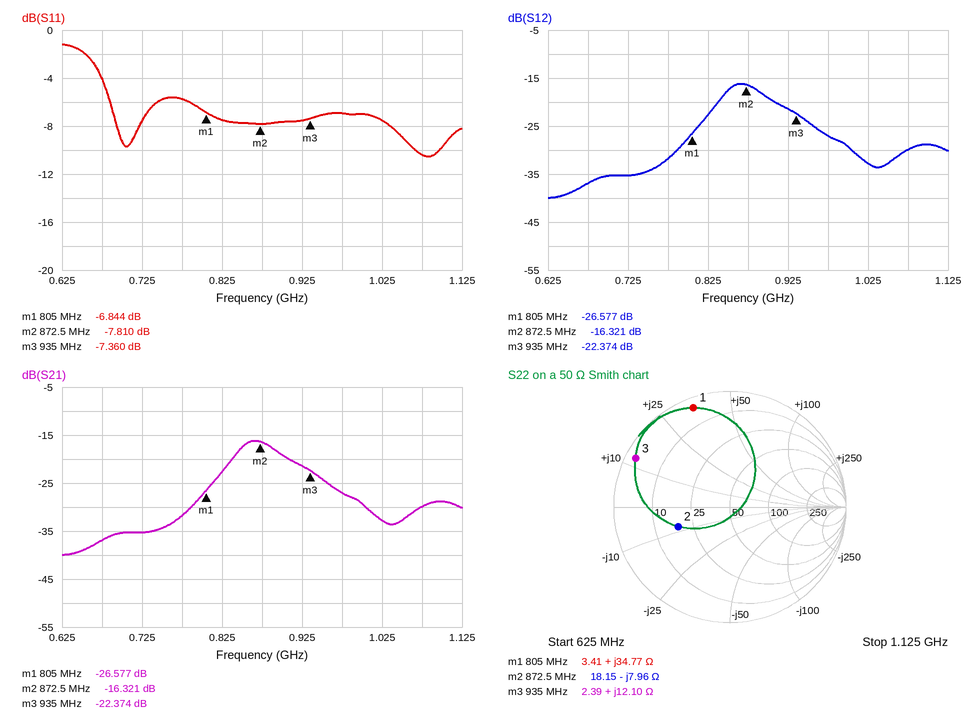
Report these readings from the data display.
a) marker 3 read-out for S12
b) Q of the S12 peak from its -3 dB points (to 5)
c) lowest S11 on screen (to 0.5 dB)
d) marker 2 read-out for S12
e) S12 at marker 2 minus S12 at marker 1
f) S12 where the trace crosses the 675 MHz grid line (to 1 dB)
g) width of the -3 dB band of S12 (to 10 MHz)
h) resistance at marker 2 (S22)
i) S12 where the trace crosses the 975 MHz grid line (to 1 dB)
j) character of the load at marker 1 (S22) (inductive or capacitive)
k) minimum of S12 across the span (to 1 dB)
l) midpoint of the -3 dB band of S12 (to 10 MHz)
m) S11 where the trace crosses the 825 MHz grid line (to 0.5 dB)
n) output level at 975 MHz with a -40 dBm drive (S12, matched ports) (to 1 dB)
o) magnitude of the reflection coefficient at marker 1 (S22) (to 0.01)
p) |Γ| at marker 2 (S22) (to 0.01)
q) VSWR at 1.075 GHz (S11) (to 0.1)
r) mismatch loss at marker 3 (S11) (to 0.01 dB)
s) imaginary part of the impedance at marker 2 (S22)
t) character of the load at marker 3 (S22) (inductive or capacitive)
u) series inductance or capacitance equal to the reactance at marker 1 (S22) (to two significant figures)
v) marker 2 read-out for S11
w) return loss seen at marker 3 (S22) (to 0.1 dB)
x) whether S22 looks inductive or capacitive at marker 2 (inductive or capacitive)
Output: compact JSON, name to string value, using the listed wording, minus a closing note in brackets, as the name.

{"marker 3 read-out for S12": "-22.374 dB", "Q of the S12 peak from its -3 dB points": "15", "lowest S11 on screen": "-10.5 dB", "marker 2 read-out for S12": "-16.321 dB", "S12 at marker 2 minus S12 at marker 1": "10.256 dB", "S12 where the trace crosses the 675 MHz grid line": "-37 dB", "width of the -3 dB band of S12": "60 MHz", "resistance at marker 2": "18.15 Ω", "S12 where the trace crosses the 975 MHz grid line": "-27 dB", "character of the load at marker 1 (S22)": "inductive", "minimum of S12 across the span": "-40 dB", "midpoint of the -3 dB band of S12": "870 MHz", "S11 where the trace crosses the 825 MHz grid line": "-7.5 dB", "output level at 975 MHz with a -40 dBm drive (S12, matched ports)": "-67 dBm", "magnitude of the reflection coefficient at marker 1 (S22)": "0.91", "|Γ| at marker 2 (S22)": "0.48", "VSWR at 1.075 GHz (S11)": "1.9", "mismatch loss at marker 3 (S11)": "0.88 dB", "imaginary part of the impedance at marker 2": "-7.96 Ω", "character of the load at marker 3 (S22)": "inductive", "series inductance or capacitance equal to the reactance at marker 1 (S22)": "6.9 nH", "marker 2 read-out for S11": "-7.810 dB", "return loss seen at marker 3 (S22)": "0.8 dB", "whether S22 looks inductive or capacitive at marker 2": "capacitive"}
